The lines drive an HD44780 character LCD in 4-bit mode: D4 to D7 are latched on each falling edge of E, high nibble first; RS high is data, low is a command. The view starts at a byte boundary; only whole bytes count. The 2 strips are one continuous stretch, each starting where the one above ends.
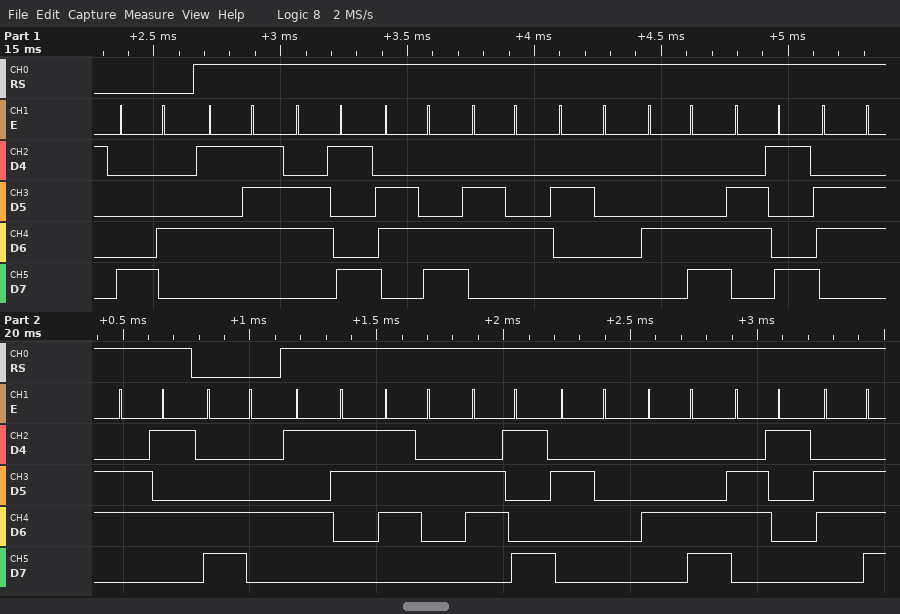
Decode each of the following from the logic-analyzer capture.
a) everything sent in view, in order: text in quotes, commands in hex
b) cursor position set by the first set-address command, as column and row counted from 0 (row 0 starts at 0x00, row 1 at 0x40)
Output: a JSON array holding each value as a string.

["0x84 \"Wild Life\" 0xC4 \"Sri Lan\"", "column 4, row 0"]
